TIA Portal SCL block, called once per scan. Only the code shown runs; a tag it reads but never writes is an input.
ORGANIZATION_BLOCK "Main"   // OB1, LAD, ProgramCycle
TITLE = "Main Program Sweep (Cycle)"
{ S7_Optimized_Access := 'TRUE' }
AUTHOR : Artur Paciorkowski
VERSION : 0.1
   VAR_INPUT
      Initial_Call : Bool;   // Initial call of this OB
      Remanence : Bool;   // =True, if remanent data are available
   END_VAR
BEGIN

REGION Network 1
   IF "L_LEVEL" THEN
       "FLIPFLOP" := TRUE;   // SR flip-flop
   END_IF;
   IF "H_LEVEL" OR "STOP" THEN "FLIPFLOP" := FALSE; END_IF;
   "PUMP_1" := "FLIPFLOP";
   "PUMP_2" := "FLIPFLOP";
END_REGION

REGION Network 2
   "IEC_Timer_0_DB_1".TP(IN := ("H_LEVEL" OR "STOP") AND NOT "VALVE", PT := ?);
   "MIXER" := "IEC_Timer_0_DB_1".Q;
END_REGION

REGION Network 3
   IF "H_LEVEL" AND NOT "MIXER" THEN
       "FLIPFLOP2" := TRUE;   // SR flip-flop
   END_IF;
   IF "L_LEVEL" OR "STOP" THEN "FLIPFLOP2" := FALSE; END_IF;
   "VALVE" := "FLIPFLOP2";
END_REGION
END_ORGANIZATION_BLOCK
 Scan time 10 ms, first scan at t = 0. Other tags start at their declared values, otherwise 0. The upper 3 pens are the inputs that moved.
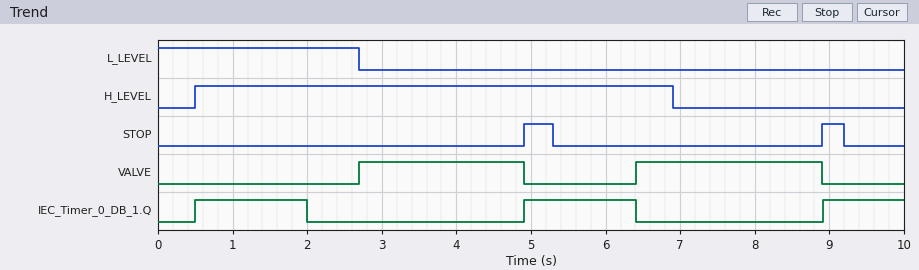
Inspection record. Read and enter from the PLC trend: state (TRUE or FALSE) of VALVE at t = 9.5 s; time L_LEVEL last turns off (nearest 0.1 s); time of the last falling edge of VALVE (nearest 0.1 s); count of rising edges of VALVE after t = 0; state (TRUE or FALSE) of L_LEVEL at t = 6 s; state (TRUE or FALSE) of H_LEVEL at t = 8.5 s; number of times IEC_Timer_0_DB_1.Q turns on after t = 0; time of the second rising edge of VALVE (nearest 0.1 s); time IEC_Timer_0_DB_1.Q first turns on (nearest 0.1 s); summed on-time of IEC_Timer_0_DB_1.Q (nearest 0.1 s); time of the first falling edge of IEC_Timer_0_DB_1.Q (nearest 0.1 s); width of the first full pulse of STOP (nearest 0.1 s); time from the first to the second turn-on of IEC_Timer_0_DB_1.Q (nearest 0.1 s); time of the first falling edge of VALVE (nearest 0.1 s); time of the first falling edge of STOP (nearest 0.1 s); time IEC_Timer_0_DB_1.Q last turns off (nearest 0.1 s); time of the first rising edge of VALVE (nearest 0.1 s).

FALSE
2.7 s
8.9 s
2
FALSE
FALSE
3
6.4 s
0.5 s
4.1 s
2.0 s
0.4 s
4.4 s
4.9 s
5.3 s
6.4 s
2.7 s
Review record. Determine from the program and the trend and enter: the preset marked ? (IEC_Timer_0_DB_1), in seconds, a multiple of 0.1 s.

1.5 s
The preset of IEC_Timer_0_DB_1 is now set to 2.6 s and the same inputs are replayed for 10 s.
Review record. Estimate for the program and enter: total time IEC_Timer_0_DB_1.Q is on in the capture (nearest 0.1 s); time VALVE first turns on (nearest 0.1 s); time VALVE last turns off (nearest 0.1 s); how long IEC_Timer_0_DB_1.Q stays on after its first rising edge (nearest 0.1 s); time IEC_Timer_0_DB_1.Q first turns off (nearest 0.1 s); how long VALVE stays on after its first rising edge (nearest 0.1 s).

6.3 s
3.1 s
4.9 s
2.6 s
3.1 s
1.8 s
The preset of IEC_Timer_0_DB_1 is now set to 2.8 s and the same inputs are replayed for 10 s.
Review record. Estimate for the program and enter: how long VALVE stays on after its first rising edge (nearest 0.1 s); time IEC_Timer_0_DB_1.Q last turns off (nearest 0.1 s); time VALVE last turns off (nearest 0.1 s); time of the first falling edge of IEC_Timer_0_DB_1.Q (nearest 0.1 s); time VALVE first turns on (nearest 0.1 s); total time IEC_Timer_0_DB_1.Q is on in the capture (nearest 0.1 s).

1.6 s
7.7 s
4.9 s
3.3 s
3.3 s
6.7 s
